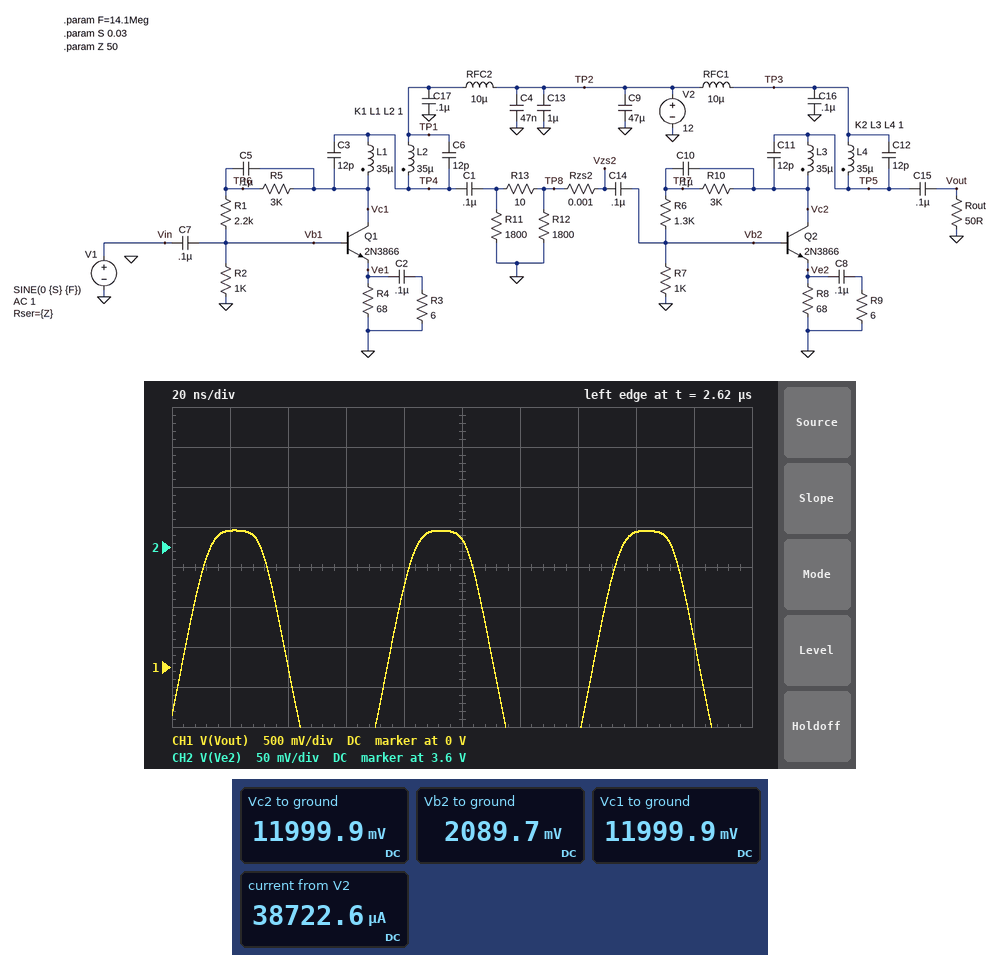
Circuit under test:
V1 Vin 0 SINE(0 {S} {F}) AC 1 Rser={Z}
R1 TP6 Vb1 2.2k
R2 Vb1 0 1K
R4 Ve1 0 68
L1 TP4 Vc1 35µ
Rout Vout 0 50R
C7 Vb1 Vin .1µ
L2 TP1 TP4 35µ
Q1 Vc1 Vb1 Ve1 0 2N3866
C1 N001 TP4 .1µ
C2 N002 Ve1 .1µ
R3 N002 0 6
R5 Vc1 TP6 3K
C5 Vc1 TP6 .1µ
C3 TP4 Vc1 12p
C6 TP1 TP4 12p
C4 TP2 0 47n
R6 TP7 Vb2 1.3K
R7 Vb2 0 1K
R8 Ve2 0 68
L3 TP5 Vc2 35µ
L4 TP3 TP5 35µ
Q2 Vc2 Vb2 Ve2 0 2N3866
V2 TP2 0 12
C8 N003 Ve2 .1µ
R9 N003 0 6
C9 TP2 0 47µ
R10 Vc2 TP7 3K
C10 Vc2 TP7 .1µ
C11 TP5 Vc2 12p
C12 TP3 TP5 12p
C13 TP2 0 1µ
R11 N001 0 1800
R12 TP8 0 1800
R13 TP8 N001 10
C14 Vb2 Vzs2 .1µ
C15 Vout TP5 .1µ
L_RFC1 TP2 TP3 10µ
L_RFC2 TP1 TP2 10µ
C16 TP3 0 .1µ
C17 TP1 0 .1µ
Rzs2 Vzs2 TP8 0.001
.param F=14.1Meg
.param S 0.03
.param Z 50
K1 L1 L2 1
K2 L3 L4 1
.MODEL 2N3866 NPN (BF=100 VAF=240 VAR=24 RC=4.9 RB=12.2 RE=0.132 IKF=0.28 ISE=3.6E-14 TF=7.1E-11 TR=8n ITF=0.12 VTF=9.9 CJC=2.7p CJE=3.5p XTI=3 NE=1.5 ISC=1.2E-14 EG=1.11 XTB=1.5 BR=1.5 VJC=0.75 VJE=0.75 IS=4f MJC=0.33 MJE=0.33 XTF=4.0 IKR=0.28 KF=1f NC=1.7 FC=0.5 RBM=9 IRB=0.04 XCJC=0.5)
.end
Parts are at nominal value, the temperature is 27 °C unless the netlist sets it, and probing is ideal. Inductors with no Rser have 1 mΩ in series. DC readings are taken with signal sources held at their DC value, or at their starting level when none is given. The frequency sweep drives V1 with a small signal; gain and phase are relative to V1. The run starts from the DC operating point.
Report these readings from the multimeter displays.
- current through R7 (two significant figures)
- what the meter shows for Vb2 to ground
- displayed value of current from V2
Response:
2.1 mA
2089.7 mV
38722.6 µA
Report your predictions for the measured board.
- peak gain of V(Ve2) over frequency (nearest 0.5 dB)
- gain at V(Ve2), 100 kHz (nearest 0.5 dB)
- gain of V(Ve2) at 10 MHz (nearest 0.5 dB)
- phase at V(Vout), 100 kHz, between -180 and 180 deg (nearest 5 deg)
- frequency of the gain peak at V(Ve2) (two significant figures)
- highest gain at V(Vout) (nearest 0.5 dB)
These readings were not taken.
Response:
19.5 dB
9.0 dB
13.0 dB
-110 deg
150 kHz
37.0 dB
